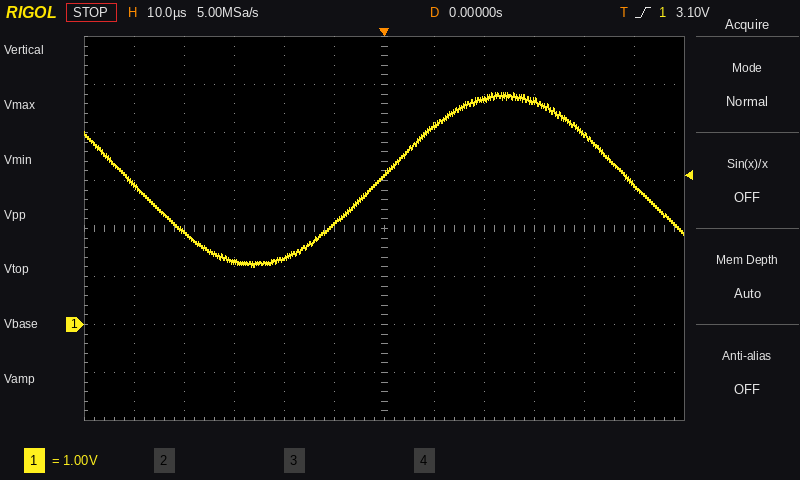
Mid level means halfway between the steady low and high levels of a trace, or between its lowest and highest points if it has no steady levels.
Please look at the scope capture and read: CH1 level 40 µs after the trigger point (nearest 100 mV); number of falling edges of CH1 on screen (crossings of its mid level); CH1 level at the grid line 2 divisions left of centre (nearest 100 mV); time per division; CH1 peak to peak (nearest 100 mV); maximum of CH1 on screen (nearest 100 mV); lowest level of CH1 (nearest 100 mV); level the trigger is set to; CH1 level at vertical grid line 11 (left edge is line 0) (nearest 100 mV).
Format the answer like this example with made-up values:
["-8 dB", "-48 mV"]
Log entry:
["4.0 V", "2", "1.4 V", "10 µs", "3.6 V", "4.8 V", "1.2 V", "3.10 V", "2.9 V"]
